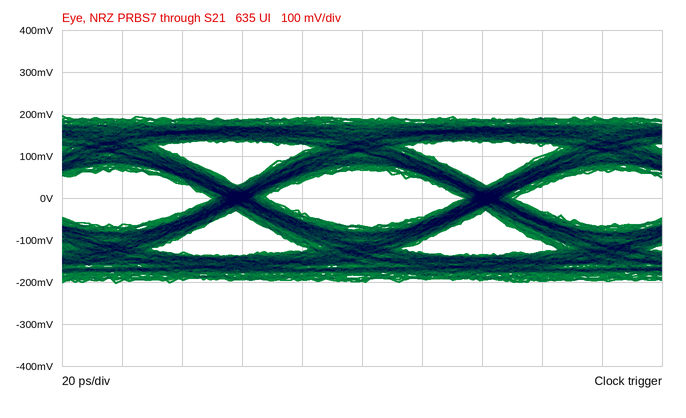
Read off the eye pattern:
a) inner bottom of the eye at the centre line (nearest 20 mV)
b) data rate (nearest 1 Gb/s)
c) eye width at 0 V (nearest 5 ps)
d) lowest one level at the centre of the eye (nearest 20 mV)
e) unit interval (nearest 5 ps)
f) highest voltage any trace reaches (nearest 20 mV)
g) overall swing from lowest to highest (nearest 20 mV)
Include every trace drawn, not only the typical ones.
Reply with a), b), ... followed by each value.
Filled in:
a) -60 mV
b) 12 Gb/s
c) 65 ps
d) 60 mV
e) 85 ps
f) 200 mV
g) 400 mV
